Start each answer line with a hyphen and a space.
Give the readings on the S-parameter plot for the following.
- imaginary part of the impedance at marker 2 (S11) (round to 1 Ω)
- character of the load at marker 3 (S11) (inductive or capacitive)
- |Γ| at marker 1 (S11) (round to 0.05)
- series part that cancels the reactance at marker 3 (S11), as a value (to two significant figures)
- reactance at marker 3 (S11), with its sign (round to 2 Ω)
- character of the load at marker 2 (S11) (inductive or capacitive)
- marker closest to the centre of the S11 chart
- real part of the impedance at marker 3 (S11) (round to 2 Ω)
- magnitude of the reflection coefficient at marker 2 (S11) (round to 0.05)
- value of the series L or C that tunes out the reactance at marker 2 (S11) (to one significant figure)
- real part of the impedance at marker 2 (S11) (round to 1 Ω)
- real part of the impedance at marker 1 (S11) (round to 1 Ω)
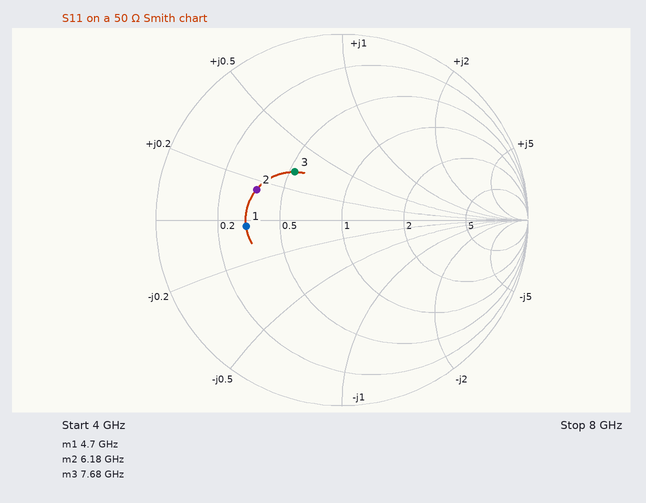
- +8 Ω
- inductive
- 0.50
- 1.3 pF
- +16 Ω
- inductive
- marker 3
- 26 Ω
- 0.50
- 3 pF
- 18 Ω
- 16 Ω
